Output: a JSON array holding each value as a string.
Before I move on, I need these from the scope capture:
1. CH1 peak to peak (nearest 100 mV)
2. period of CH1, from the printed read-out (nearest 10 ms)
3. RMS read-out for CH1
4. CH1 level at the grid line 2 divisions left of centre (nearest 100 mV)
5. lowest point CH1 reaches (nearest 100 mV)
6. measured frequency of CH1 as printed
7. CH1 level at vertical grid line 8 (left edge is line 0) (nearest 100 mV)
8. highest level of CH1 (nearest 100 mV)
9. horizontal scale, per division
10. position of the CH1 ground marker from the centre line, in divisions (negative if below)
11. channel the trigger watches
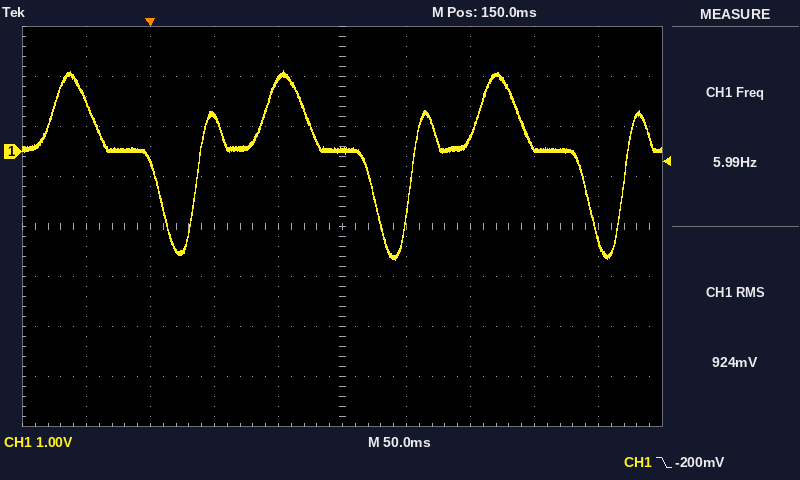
["3.8 V", "170 ms", "924 mV", "700 mV", "-2.2 V", "5.99 Hz", "100 mV", "1.6 V", "50 ms", "+1.5 div", "CH1"]
